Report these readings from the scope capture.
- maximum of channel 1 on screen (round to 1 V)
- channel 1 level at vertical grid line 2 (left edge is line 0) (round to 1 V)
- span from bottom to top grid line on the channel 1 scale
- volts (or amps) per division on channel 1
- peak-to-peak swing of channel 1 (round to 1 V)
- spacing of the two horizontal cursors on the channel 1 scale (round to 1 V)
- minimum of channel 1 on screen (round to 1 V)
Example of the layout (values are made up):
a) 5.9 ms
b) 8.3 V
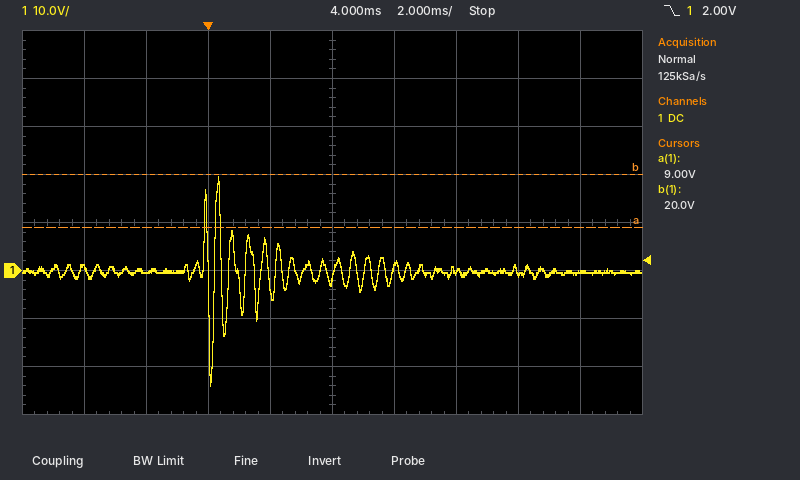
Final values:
a) 20 V
b) 0 V
c) 80 V
d) 10 V
e) 44 V
f) 11 V
g) -24 V
